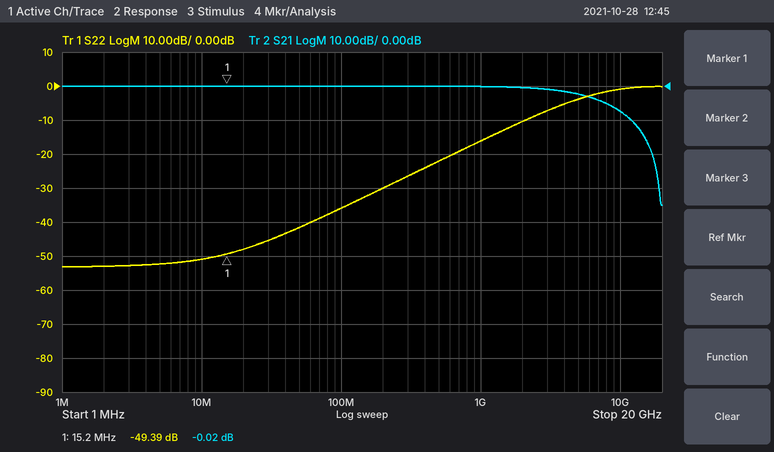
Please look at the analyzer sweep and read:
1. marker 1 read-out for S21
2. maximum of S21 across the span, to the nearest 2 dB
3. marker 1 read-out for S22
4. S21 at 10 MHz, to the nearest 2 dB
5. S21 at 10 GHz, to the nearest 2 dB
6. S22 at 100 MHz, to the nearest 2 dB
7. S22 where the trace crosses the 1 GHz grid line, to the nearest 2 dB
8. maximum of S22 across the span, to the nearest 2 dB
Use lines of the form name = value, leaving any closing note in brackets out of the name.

marker 1 read-out for S21 = -0.02 dB
maximum of S21 across the span, to the nearest 2 dB = 0 dB
marker 1 read-out for S22 = -49.39 dB
S21 at 10 MHz, to the nearest 2 dB = 0 dB
S21 at 10 GHz, to the nearest 2 dB = -8 dB
S22 at 100 MHz, to the nearest 2 dB = -36 dB
S22 where the trace crosses the 1 GHz grid line, to the nearest 2 dB = -16 dB
maximum of S22 across the span, to the nearest 2 dB = 0 dB
